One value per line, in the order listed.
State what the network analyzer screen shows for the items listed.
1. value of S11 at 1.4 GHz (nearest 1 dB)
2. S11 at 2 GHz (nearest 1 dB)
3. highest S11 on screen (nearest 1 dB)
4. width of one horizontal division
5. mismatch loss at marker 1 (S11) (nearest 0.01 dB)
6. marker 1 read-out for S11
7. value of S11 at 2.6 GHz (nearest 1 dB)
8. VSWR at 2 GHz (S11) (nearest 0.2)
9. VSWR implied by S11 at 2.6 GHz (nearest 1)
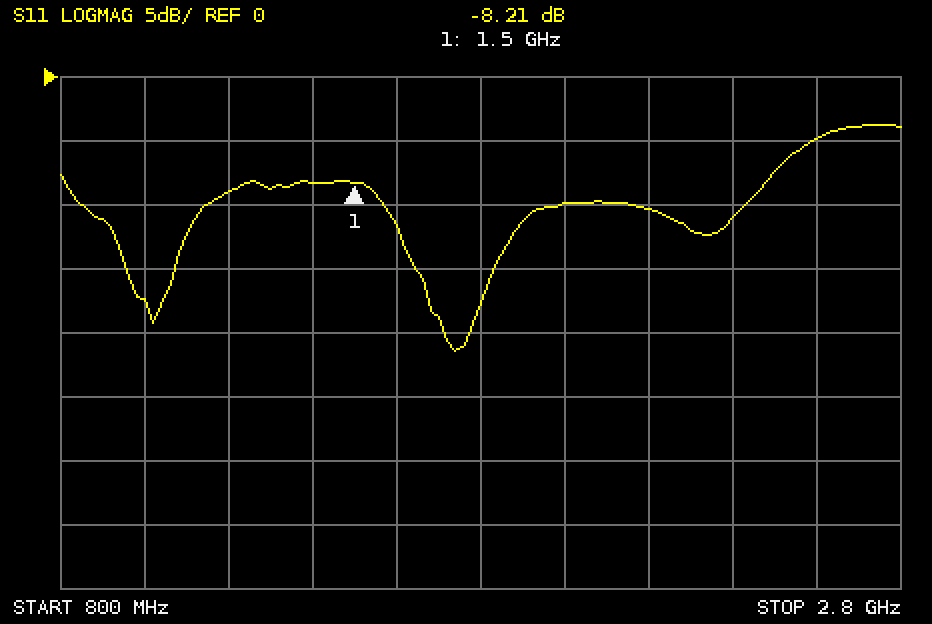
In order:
-8 dB
-10 dB
-4 dB
200 MHz
0.71 dB
-8.21 dB
-5 dB
2.0
4
